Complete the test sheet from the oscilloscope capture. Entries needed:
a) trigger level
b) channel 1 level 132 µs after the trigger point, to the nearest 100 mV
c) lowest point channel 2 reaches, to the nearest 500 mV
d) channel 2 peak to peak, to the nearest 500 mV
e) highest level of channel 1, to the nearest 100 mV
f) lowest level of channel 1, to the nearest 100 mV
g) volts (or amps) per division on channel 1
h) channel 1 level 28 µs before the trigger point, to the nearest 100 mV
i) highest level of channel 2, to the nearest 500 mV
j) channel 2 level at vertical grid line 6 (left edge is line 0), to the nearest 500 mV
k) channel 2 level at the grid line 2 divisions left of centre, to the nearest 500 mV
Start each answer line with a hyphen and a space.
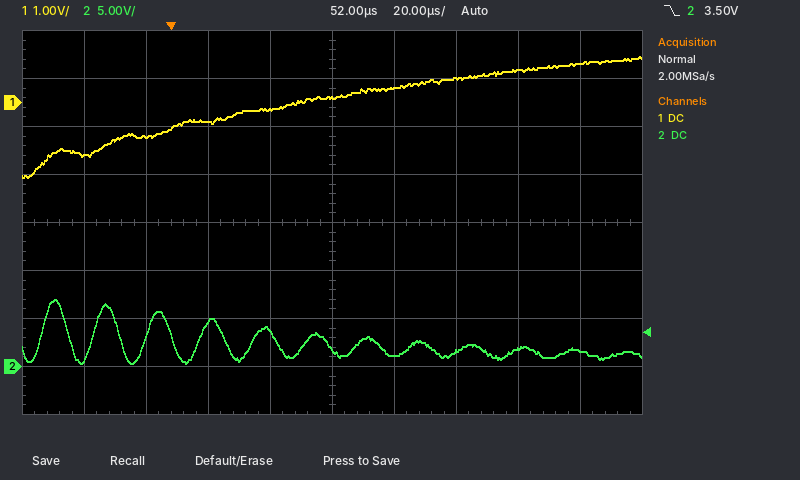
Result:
- 3.50 V
- 800 mV
- 500 mV
- 6.5 V
- 1.0 V
- -1.6 V
- 1 V
- -1.1 V
- 7.0 V
- 1.0 V
- 4.5 V
